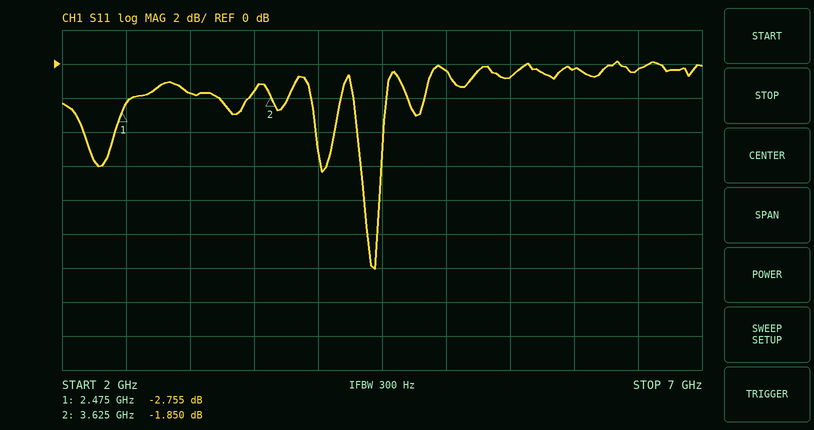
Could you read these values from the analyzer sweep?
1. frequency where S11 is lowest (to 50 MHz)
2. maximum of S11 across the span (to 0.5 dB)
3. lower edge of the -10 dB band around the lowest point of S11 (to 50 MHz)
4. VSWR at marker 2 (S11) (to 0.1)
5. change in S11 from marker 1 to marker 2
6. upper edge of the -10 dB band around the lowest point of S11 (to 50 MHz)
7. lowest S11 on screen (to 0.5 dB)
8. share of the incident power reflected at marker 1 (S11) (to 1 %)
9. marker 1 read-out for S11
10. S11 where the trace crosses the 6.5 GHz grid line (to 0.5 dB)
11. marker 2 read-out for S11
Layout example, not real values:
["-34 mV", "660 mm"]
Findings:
["4.45 GHz", "0.0 dB", "4.40 GHz", "9.4", "0.905 dB", "4.45 GHz", "-12.0 dB", "53 %", "-2.755 dB", "-0.5 dB", "-1.850 dB"]
